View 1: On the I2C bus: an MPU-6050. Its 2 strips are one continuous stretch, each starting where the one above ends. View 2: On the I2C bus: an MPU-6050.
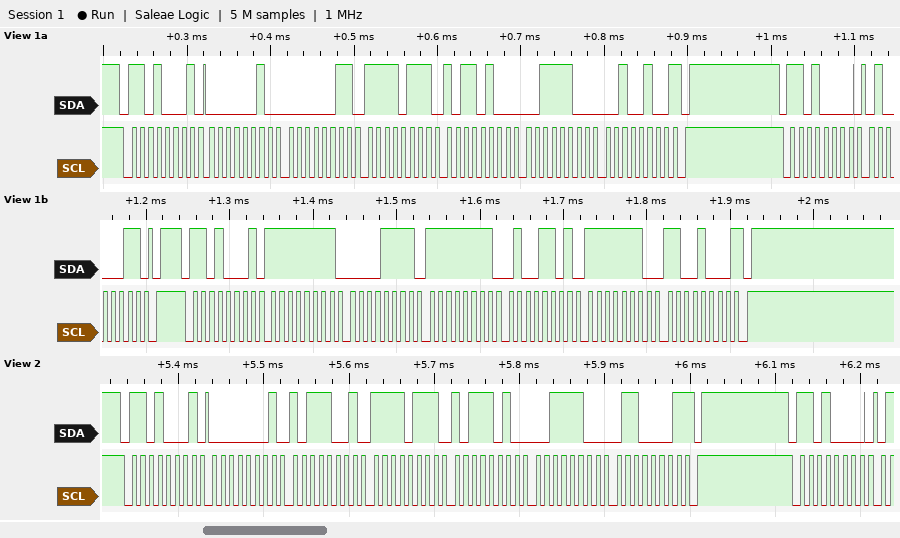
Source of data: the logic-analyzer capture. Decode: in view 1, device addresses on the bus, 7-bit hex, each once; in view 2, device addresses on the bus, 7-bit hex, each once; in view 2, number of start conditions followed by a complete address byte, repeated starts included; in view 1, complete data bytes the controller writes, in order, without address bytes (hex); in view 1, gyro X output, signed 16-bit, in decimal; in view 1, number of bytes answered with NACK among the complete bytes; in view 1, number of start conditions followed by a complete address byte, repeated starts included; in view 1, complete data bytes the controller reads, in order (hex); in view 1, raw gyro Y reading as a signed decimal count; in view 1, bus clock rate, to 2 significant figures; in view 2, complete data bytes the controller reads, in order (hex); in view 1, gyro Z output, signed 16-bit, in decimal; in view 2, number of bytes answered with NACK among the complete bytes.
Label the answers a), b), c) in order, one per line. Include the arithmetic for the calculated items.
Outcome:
a) 0x68
b) 0x68
c) 2
d) 43
e) 0xFF0F = -241
f) 2
g) 3
h) 02 03 F7 B4 3C 24 FF 0F FF 4D FE C8
i) 0xFF4D = -179
j) 100 kHz
k) 01 B9 F7 BA 3C 61
l) 0xFEC8 = -312
m) 1
